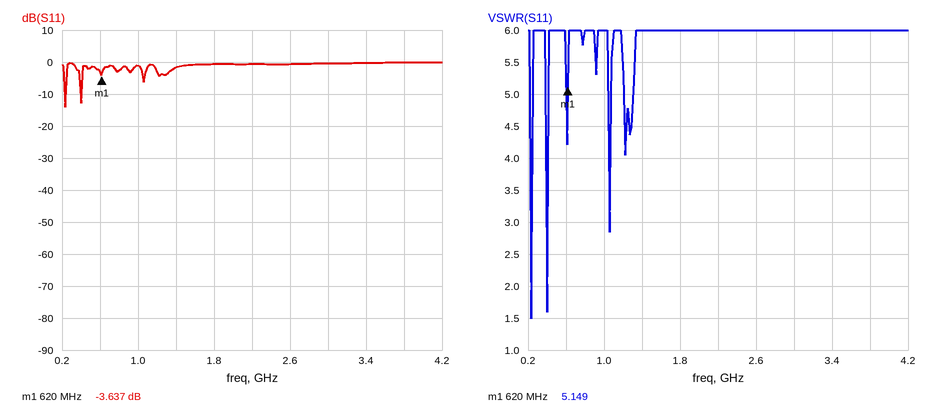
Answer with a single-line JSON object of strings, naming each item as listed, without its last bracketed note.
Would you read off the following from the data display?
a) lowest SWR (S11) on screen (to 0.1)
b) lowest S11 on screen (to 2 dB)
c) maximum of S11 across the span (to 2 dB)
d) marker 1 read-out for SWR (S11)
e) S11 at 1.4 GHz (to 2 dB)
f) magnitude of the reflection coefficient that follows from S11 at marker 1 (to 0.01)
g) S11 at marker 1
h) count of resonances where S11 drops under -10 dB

{"lowest SWR (S11) on screen": "1.5", "lowest S11 on screen": "-14 dB", "maximum of S11 across the span": "0 dB", "marker 1 read-out for SWR": "5.149", "S11 at 1.4 GHz": "-2 dB", "magnitude of the reflection coefficient that follows from S11 at marker 1": "0.66", "S11 at marker 1": "-3.637 dB", "count of resonances where S11 drops under -10 dB": "2"}
